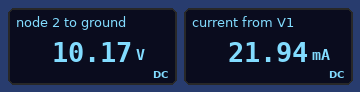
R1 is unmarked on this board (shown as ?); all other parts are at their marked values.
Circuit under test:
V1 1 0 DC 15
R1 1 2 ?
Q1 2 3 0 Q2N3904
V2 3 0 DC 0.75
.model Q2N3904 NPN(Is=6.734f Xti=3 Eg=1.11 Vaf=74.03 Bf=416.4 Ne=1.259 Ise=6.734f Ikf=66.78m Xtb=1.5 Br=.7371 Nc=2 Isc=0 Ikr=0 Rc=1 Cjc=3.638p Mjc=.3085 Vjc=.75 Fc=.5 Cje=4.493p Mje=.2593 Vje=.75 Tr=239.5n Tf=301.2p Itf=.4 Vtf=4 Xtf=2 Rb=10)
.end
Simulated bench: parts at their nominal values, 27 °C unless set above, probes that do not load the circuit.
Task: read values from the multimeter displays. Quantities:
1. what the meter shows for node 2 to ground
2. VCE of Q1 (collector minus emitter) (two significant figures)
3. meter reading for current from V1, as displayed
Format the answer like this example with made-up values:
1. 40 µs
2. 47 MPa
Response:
1. 10.17 V
2. 10 V
3. 21.94 mA
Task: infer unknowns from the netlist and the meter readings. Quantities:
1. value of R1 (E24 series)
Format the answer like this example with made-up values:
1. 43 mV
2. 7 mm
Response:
1. 220 Ω
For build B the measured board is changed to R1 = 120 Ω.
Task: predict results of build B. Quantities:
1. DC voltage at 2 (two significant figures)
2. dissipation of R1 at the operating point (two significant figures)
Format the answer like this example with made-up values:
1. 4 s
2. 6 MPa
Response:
1. 12 V
2. 61 mW
